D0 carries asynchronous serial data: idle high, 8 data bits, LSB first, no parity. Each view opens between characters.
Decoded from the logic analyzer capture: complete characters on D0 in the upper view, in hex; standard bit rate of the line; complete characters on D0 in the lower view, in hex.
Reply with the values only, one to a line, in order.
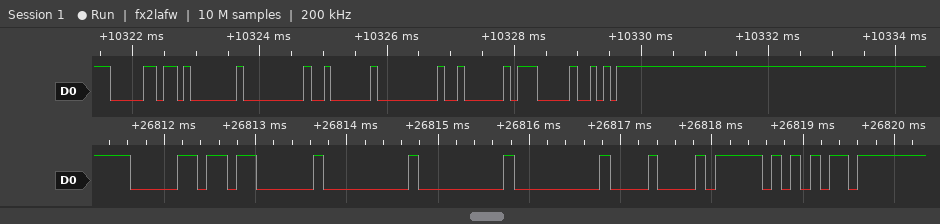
B0, 01, 00, 02, 00, 02, 07, EA
9600 baud
B0, 03, 00, 00, 00, 08, 5F, ED
